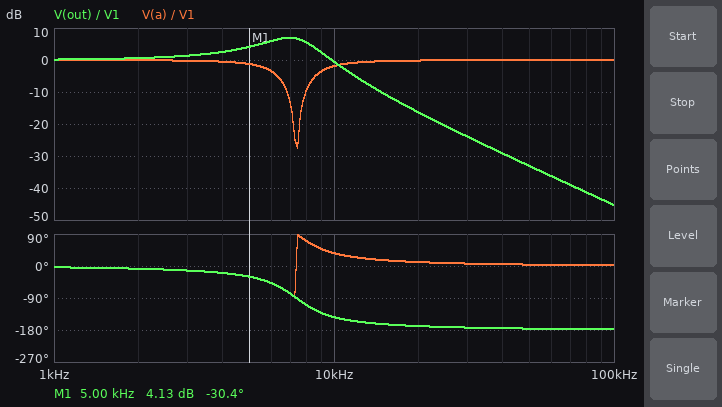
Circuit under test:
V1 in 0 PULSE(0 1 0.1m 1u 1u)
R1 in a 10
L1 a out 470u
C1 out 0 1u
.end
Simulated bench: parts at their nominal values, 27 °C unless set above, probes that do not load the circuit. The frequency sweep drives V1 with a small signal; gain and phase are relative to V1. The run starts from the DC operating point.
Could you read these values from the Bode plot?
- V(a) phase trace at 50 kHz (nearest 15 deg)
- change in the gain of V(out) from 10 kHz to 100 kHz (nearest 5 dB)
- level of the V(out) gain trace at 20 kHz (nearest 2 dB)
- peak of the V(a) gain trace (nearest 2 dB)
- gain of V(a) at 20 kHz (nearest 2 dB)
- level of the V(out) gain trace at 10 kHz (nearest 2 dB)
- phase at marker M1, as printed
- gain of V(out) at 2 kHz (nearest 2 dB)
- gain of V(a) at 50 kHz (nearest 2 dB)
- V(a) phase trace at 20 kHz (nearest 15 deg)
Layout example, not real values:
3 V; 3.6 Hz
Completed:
0 deg; -45 dB; -16 dB; 0 dB; 0 dB; 0 dB; -30.4 deg; 0 dB; 0 dB; 15 deg
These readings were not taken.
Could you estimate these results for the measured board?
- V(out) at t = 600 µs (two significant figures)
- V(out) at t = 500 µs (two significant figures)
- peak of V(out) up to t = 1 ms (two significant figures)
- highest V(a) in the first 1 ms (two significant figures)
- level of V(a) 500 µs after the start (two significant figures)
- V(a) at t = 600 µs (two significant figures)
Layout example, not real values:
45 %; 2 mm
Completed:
1.0 V; 990 mV; 1.5 V; 1.2 V; 1.0 V; 1.0 V
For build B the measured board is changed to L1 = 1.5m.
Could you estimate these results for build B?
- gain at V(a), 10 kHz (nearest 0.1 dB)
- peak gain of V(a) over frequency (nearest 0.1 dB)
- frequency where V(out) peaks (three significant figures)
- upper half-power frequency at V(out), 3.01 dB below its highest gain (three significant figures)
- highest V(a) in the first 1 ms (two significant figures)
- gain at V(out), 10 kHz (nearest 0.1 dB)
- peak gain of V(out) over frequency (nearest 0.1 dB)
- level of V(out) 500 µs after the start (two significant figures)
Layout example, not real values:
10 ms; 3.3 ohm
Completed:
-0.1 dB; 0 dB; 4.04 kHz; 4.54 kHz; 1.1 V; -13.9 dB; 11.8 dB; 1.2 V
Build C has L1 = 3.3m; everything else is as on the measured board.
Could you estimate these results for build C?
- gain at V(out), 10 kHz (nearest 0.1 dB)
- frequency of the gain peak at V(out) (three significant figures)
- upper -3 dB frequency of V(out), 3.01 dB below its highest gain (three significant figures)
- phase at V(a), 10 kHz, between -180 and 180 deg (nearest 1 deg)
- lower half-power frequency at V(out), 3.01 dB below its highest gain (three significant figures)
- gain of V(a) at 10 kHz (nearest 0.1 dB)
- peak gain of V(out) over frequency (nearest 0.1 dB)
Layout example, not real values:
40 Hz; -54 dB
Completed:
-21.6 dB; 2.75 kHz; 2.98 kHz; 3 deg; 2.50 kHz; 0 dB; 15.2 dB
